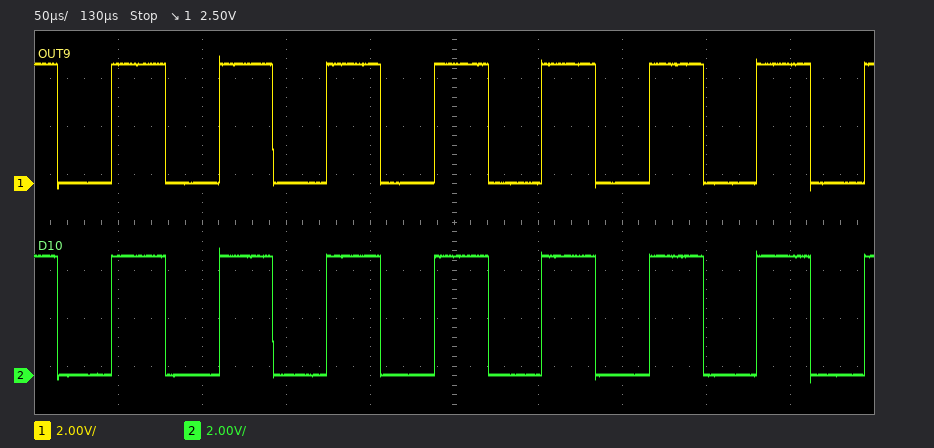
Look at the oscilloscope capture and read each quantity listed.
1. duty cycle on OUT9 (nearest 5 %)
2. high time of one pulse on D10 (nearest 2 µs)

50 %
32 µs
